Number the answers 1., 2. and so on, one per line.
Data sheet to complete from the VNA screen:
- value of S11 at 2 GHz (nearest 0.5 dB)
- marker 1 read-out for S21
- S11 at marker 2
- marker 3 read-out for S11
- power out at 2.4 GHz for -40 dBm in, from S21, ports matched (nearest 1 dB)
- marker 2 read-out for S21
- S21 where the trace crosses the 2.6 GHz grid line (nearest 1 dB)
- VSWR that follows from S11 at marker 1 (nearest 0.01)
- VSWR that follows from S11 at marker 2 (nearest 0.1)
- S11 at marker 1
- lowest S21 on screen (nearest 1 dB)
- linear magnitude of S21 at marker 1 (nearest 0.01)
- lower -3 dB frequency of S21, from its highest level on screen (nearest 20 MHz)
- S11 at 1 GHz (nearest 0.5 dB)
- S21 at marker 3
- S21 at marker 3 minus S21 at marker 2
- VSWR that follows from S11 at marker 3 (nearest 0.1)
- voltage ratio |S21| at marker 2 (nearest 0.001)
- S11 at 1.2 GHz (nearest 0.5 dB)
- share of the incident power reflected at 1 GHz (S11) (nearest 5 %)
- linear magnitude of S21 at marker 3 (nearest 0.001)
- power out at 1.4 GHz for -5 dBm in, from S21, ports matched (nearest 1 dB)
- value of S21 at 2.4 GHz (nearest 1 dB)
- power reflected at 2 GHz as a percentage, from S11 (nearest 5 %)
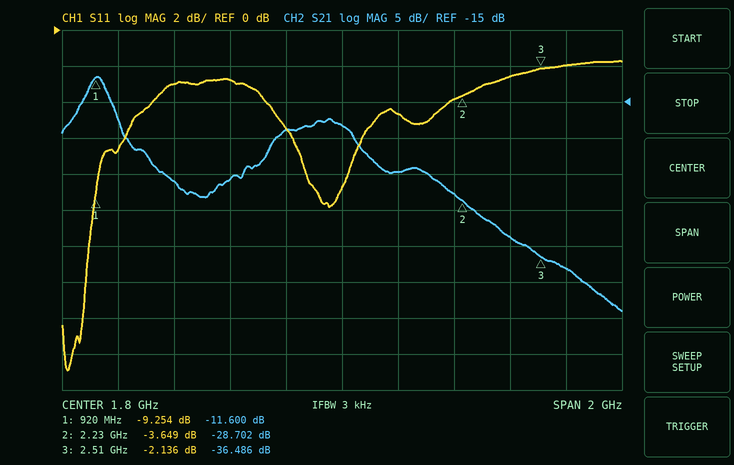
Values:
1. -4.5 dB
2. -11.600 dB
3. -3.649 dB
4. -2.136 dB
5. -74 dBm
6. -28.702 dB
7. -38 dB
8. 2.05
9. 4.8
10. -9.254 dB
11. -44 dB
12. 0.26
13. 880 MHz
14. -6.5 dB
15. -36.486 dB
16. -7.784 dB
17. 8.2
18. 0.037
19. -3.0 dB
20. 20 %
21. 0.015
22. -31 dBm
23. -34 dB
24. 35 %
